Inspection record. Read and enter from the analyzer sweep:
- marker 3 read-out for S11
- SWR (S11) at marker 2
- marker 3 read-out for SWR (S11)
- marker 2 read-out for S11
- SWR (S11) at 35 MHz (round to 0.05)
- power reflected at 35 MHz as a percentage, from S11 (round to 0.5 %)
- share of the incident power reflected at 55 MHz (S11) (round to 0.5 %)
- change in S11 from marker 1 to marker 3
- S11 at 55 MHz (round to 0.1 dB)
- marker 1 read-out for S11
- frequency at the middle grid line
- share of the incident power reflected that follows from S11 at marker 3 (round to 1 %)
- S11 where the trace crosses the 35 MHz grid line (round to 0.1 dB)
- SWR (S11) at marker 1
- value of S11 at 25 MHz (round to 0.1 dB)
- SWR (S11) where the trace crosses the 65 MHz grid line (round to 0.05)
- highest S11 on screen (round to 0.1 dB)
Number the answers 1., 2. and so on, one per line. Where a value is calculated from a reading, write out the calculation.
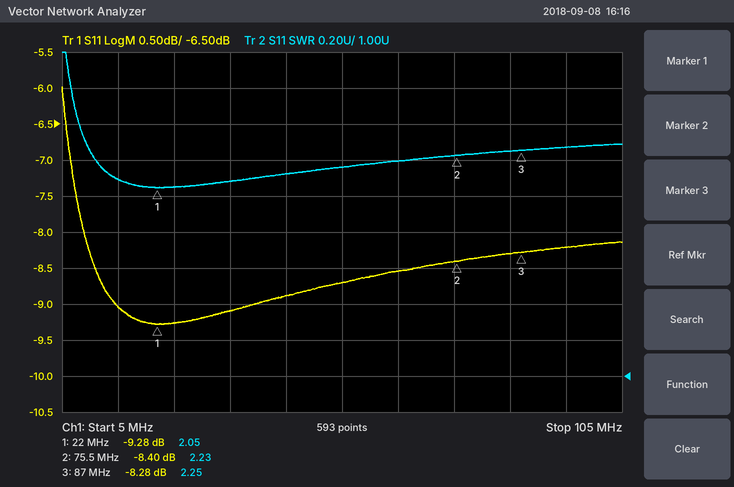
1. -8.28 dB
2. 2.23
3. 2.25
4. -8.40 dB
5. 2.10
6. 10^(-9.1/10) ≈ 12.3 %, so 12.5 % to the nearest 0.5 %
7. 10^(-8.7/10) ≈ 13.5 %
8. -8.28 − (-9.28) = 1.00 dB
9. -8.7 dB
10. -9.28 dB
11. 55 MHz
12. 10^(-8.28/10) ≈ 15 %
13. -9.1 dB
14. 2.05
15. -9.3 dB
16. 2.20
17. -6.0 dB
